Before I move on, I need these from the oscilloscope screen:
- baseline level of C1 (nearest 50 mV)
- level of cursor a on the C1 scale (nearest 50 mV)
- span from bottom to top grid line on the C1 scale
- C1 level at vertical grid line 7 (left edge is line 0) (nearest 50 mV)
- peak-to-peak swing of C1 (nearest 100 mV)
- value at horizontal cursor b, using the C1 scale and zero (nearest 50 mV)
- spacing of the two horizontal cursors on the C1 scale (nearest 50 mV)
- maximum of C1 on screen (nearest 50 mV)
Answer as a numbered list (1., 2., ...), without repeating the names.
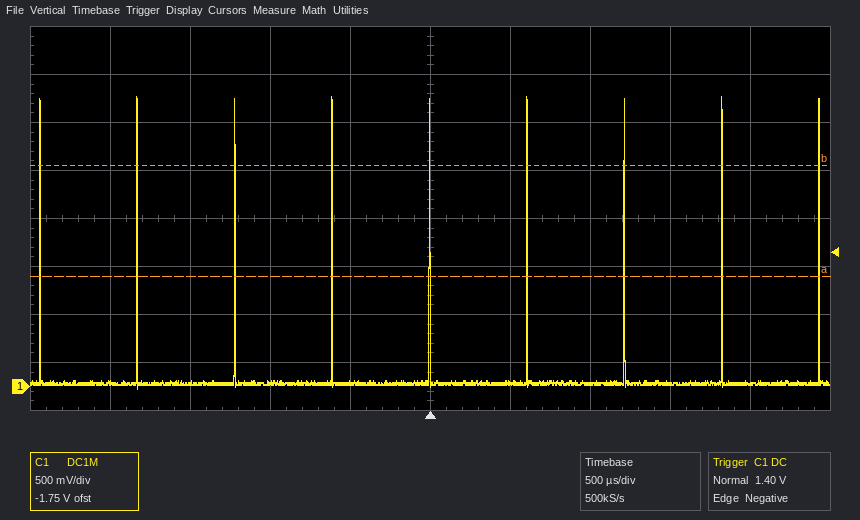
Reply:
1. 50 mV
2. 1.15 V
3. 4 V
4. 50 mV
5. 3.00 V
6. 2.30 V
7. 1.15 V
8. 3.00 V
